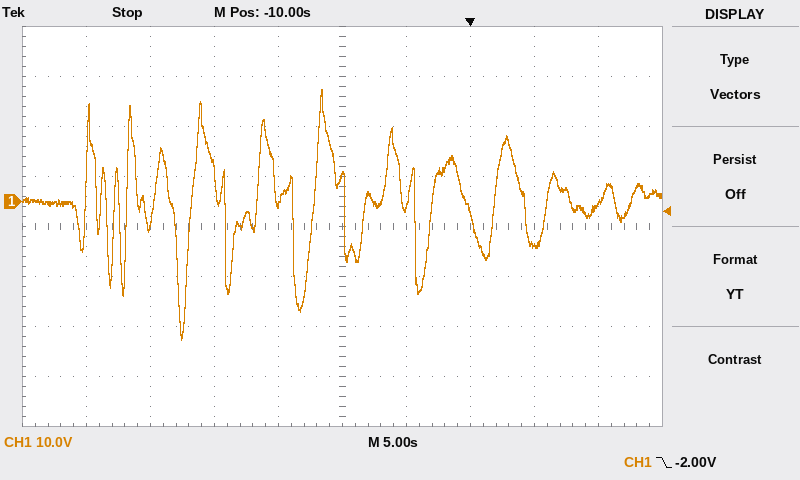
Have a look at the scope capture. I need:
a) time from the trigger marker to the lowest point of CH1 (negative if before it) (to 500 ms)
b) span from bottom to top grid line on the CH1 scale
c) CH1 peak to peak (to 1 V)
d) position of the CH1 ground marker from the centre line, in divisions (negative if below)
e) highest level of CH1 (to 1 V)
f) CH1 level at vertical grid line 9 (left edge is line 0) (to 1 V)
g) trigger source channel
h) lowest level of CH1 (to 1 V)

-22.5 s
80 V
50 V
+0.5 div
22 V
0 V
CH1
-28 V
